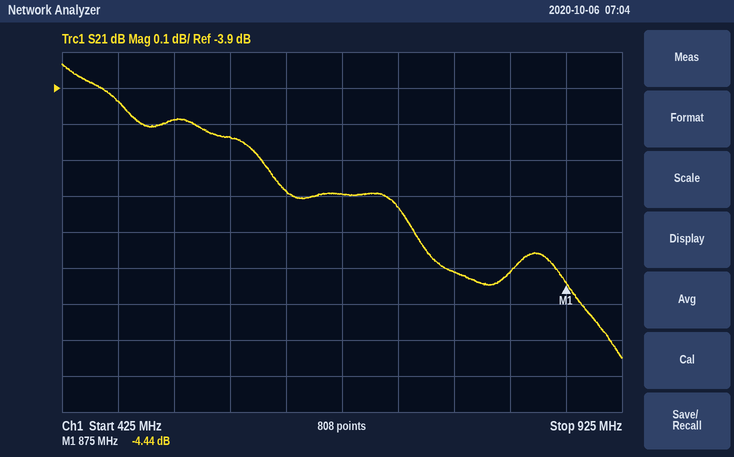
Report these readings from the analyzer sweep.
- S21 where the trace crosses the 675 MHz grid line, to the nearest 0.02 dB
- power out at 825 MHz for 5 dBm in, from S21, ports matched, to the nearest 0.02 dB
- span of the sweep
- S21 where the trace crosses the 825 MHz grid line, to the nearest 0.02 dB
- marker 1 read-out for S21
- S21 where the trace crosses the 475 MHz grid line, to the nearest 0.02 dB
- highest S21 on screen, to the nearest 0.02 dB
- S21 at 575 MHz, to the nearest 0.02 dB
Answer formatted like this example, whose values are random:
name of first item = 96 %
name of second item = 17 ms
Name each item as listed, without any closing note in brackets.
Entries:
S21 where the trace crosses the 675 MHz grid line, to the nearest 0.02 dB = -4.20 dB
power out at 825 MHz for 5 dBm in, from S21, ports matched, to the nearest 0.02 dB = 0.58 dBm
span of the sweep = 500 MHz
S21 where the trace crosses the 825 MHz grid line, to the nearest 0.02 dB = -4.42 dB
marker 1 read-out for S21 = -4.44 dB
S21 where the trace crosses the 475 MHz grid line, to the nearest 0.02 dB = -3.94 dB
highest S21 on screen, to the nearest 0.02 dB = -3.84 dB
S21 at 575 MHz, to the nearest 0.02 dB = -4.04 dB
